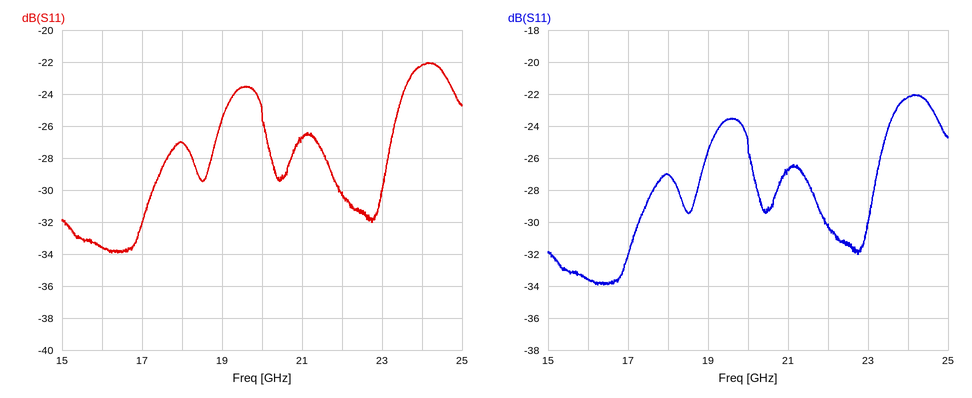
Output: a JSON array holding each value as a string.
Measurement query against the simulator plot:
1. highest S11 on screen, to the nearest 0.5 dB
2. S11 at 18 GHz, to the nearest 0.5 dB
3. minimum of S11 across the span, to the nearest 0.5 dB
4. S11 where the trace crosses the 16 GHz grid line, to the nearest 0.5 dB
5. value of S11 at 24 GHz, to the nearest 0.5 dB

["-22.0 dB", "-27.0 dB", "-34.0 dB", "-33.5 dB", "-22.0 dB"]
